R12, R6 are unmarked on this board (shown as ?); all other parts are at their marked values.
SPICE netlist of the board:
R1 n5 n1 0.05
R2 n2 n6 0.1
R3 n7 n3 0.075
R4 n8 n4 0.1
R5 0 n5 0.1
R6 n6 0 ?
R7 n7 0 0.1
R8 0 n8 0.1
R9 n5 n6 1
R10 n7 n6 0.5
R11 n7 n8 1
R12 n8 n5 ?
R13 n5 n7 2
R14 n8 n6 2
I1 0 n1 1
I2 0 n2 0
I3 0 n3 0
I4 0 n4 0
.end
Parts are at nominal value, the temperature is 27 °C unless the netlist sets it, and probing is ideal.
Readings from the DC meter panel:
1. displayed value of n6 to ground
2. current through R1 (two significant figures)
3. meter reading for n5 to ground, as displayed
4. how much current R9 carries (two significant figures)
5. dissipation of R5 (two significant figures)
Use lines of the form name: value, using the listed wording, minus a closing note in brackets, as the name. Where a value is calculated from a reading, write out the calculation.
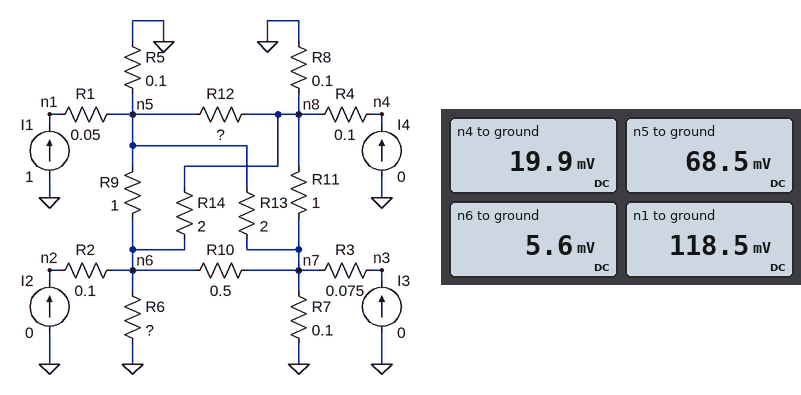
displayed value of n6 to ground: 5.6 mV
current through R1: (118.5 mV - 68.5 mV) / 50 mΩ = 1.0 A
meter reading for n5 to ground, as displayed: 68.5 mV
how much current R9 carries: (68.5 mV - 5.6 mV) / 1 Ω = 63 mA
dissipation of R5: (68.5 mV)^2 / 100 mΩ = 47 mW
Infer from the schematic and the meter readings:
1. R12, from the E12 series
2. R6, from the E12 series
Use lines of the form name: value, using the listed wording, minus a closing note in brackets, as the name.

R12, from the E12 series: 0.22 Ω
R6, from the E12 series: 0.082 Ω
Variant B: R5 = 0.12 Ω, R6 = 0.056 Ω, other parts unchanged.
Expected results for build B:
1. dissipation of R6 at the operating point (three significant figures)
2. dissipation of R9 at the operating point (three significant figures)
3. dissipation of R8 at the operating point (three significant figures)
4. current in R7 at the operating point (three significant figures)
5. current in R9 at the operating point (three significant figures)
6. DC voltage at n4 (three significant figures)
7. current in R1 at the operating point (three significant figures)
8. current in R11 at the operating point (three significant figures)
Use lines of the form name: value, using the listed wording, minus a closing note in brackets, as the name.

dissipation of R6 at the operating point: 381 µW
dissipation of R9 at the operating point: 5.25 mW
dissipation of R8 at the operating point: 4.98 mW
current in R7 at the operating point: 51.9 mA
current in R9 at the operating point: 72.5 mA
DC voltage at n4: 22.3 mV
current in R1 at the operating point: 1.00 A
current in R11 at the operating point: 17.1 mA
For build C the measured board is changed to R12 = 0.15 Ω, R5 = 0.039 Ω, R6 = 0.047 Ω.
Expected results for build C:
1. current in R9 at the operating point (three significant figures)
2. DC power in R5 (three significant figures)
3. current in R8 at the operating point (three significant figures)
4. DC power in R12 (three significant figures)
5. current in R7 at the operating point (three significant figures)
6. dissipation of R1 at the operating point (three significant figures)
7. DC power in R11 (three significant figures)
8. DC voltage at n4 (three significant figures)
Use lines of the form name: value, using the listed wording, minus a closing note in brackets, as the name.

current in R9 at the operating point: 30.3 mA
DC power in R5: 26.3 mW
current in R8 at the operating point: 119 mA
DC power in R12: 2.69 mW
current in R7 at the operating point: 23.2 mA
dissipation of R1 at the operating point: 50.0 mW
DC power in R11: 92.2 µW
DC voltage at n4: 11.9 mV
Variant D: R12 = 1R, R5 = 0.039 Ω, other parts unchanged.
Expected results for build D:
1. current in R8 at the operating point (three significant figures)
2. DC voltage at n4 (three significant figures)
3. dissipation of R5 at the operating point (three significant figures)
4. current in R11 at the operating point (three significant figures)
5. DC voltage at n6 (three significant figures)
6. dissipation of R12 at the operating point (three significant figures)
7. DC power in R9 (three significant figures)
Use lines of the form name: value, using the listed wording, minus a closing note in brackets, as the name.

current in R8 at the operating point: 31.2 mA
DC voltage at n4: 3.12 mV
dissipation of R5 at the operating point: 32.8 mW
current in R11 at the operating point: 1.18 mA
DC voltage at n6: 2.63 mV
dissipation of R12 at the operating point: 1.07 mW
DC power in R9: 1.10 mW
